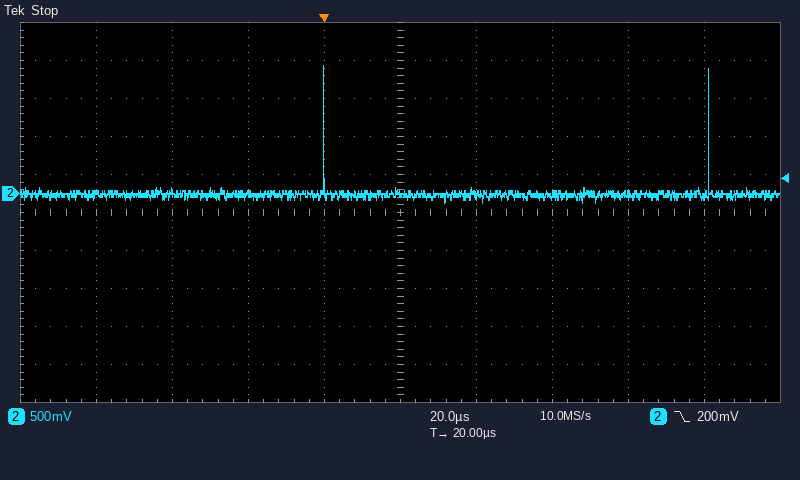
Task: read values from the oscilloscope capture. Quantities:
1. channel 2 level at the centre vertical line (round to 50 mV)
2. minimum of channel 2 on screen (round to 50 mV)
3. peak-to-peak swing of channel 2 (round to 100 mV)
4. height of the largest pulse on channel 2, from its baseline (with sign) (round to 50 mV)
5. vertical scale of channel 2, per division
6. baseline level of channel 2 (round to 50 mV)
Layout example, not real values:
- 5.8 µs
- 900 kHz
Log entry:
- 0 mV
- -100 mV
- 1.80 V
- +1.70 V
- 500 mV
- 0 mV
